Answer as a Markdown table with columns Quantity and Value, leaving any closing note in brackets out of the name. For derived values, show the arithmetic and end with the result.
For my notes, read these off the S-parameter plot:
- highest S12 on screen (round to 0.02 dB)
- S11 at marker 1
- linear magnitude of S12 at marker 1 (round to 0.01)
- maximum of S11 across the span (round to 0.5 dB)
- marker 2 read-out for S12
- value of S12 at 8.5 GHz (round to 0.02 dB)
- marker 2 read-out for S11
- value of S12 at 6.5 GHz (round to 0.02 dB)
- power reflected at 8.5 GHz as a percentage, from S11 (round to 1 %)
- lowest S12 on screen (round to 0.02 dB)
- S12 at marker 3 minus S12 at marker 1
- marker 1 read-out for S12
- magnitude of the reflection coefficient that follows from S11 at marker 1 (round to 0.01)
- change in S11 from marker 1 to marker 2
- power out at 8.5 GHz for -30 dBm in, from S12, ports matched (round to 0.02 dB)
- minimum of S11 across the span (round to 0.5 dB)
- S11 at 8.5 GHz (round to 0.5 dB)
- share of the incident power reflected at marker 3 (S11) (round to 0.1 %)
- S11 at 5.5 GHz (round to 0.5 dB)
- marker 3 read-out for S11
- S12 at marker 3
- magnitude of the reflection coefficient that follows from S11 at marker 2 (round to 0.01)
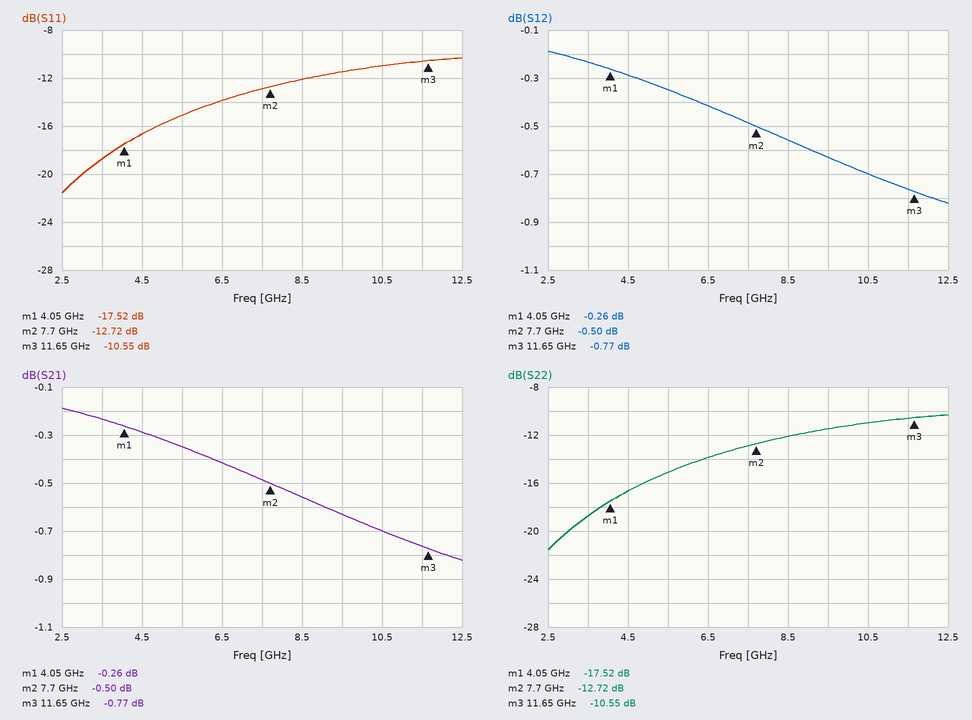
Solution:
| Quantity | Value |
|---|---|
| highest S12 on screen | -0.18 dB |
| S11 at marker 1 | -17.52 dB |
| linear magnitude of S12 at marker 1 | 10^(-0.26/20) ≈ 0.97 |
| maximum of S11 across the span | -10.5 dB |
| marker 2 read-out for S12 | -0.50 dB |
| value of S12 at 8.5 GHz | -0.56 dB |
| marker 2 read-out for S11 | -12.72 dB |
| value of S12 at 6.5 GHz | -0.42 dB |
| power reflected at 8.5 GHz as a percentage, from S11 | 10^(-12/10) ≈ 6 % |
| lowest S12 on screen | -0.82 dB |
| S12 at marker 3 minus S12 at marker 1 | -0.77 − (-0.26) = -0.51 dB |
| marker 1 read-out for S12 | -0.26 dB |
| magnitude of the reflection coefficient that follows from S11 at marker 1 | 10^(-17.52/20) ≈ 0.13 |
| change in S11 from marker 1 to marker 2 | -12.72 − (-17.52) = 4.80 dB |
| power out at 8.5 GHz for -30 dBm in, from S12, ports matched | -30 dBm + (-0.56 dB) = -30.56 dBm |
| minimum of S11 across the span | -21.5 dB |
| S11 at 8.5 GHz | -12.0 dB |
| share of the incident power reflected at marker 3 (S11) | 10^(-10.55/10) ≈ 8.8 % |
| S11 at 5.5 GHz | -15.0 dB |
| marker 3 read-out for S11 | -10.55 dB |
| S12 at marker 3 | -0.77 dB |
| magnitude of the reflection coefficient that follows from S11 at marker 2 | 10^(-12.72/20) ≈ 0.23 |
